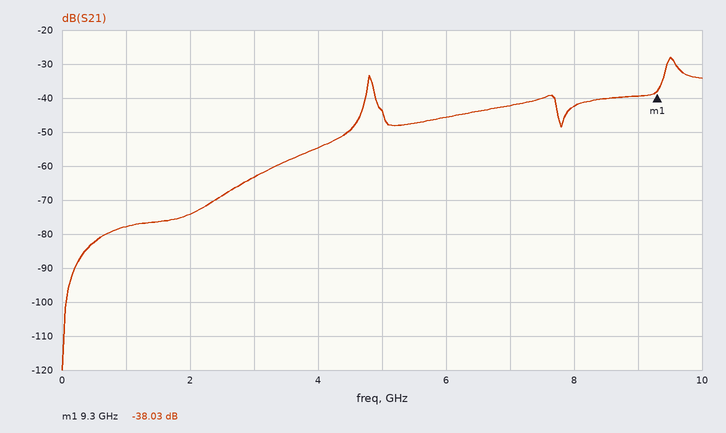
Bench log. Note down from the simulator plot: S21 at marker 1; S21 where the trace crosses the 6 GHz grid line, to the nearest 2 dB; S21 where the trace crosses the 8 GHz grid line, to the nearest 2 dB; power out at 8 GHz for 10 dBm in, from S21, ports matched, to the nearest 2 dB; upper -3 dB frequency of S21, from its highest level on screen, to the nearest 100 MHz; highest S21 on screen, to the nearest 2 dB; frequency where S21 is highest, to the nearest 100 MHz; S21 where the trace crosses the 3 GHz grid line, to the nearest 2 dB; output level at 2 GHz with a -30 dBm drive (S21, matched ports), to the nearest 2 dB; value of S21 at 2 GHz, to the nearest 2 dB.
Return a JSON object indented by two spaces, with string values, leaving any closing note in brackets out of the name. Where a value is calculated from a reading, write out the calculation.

{
  "S21 at marker 1": "-38.03 dB",
  "S21 where the trace crosses the 6 GHz grid line, to the nearest 2 dB": "-46 dB",
  "S21 where the trace crosses the 8 GHz grid line, to the nearest 2 dB": "-42 dB",
  "power out at 8 GHz for 10 dBm in, from S21, ports matched, to the nearest 2 dB": "10 dBm + (-42 dB) = -32 dBm",
  "upper -3 dB frequency of S21, from its highest level on screen, to the nearest 100 MHz": "9.6 GHz",
  "highest S21 on screen, to the nearest 2 dB": "-28 dB",
  "frequency where S21 is highest, to the nearest 100 MHz": "9.5 GHz",
  "S21 where the trace crosses the 3 GHz grid line, to the nearest 2 dB": "-64 dB",
  "output level at 2 GHz with a -30 dBm drive (S21, matched ports), to the nearest 2 dB": "-30 dBm + (-74 dB) = -104 dBm",
  "value of S21 at 2 GHz, to the nearest 2 dB": "-74 dB"
}
